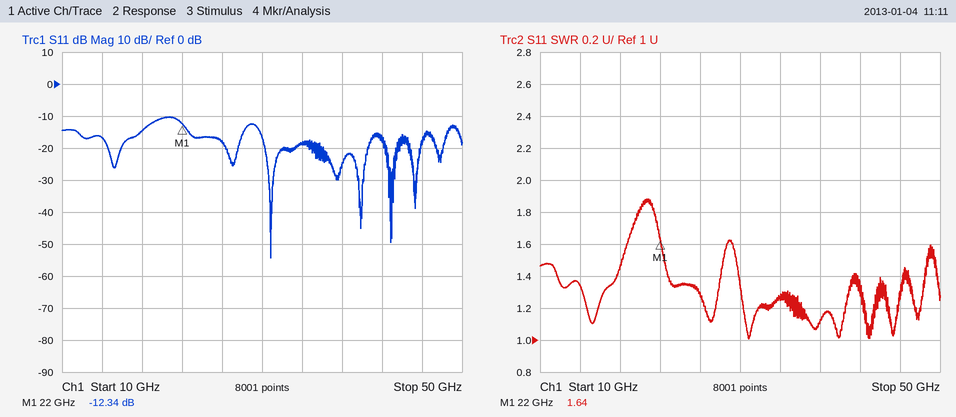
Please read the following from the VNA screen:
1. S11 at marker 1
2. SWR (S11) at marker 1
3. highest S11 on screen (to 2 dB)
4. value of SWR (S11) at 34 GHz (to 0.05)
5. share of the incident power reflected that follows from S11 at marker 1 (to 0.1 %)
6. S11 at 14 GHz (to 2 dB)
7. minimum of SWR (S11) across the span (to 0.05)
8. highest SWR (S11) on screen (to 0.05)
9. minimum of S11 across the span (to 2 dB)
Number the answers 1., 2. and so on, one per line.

1. -12.34 dB
2. 1.64
3. -10 dB
4. 1.25
5. 5.8 %
6. -16 dB
7. 1.00
8. 1.90
9. -54 dB
